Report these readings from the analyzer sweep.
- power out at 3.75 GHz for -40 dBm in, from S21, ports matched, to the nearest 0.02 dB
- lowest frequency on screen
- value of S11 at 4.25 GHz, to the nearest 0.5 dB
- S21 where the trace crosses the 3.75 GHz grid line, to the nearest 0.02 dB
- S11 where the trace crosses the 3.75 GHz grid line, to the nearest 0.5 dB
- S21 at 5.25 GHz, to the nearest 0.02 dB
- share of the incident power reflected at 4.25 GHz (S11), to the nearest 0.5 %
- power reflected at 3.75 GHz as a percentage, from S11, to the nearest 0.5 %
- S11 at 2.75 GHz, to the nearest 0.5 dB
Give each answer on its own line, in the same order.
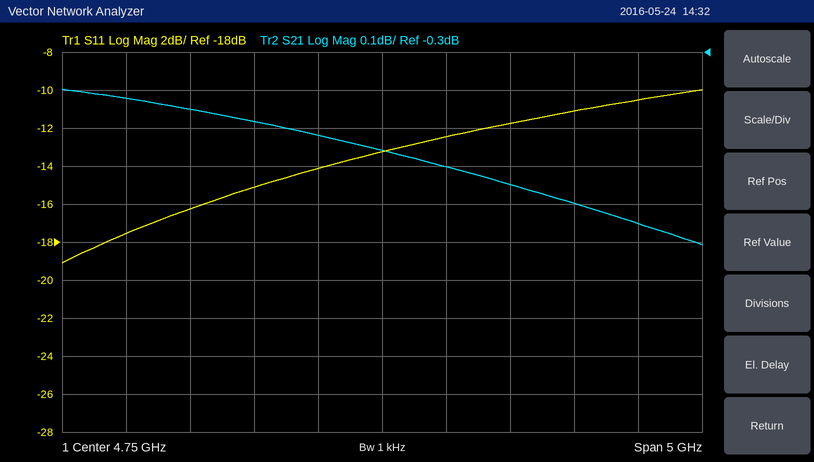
-40.48 dBm
2.25 GHz
-14.0 dB
-0.48 dB
-15.0 dB
-0.60 dB
4.0 %
3.0 %
-17.5 dB
